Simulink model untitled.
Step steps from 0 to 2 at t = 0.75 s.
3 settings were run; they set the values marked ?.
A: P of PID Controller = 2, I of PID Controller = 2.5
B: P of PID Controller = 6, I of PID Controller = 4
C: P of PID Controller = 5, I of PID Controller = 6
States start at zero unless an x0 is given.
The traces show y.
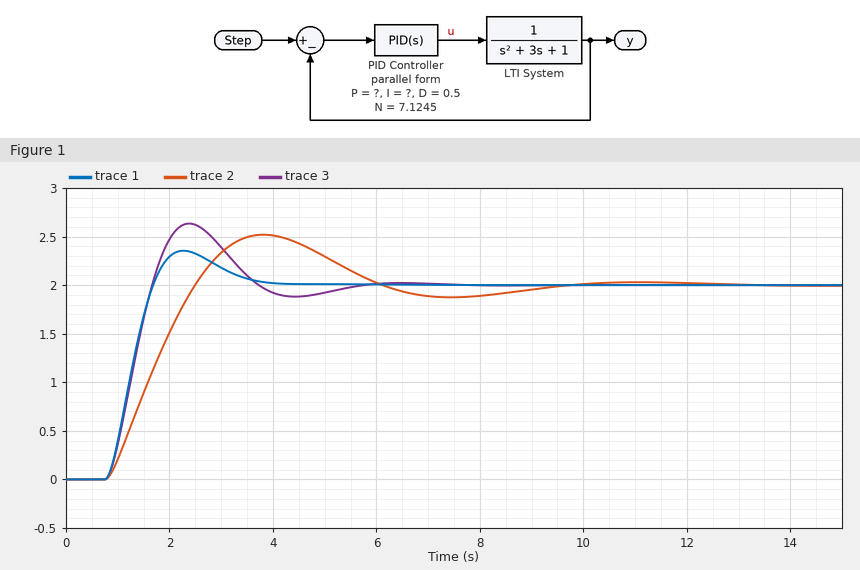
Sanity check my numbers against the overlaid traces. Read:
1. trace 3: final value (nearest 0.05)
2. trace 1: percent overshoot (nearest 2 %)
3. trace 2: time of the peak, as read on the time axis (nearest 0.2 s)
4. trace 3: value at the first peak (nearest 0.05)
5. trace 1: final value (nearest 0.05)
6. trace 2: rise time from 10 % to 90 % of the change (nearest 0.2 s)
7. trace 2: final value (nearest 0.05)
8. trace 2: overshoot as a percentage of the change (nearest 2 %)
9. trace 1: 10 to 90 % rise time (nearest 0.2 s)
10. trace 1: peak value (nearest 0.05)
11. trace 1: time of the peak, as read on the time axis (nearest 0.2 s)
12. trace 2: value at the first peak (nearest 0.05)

2.00
18 %
3.8 s
2.65
2.00
1.2 s
2.00
26 %
0.6 s
2.35
2.2 s
2.50
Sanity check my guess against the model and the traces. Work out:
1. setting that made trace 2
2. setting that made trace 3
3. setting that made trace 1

A
C
B
